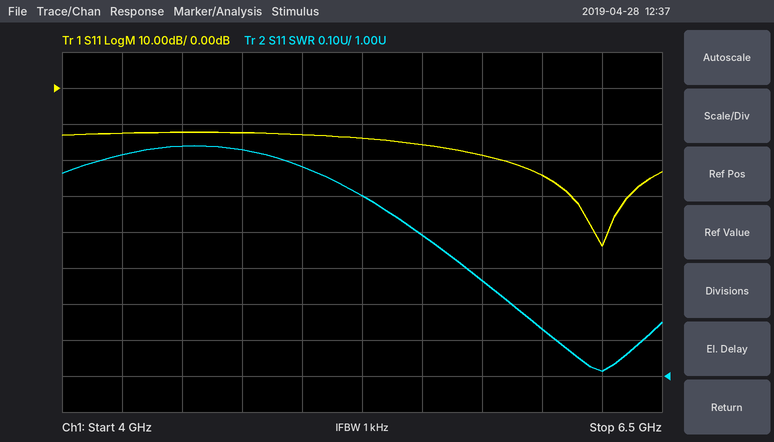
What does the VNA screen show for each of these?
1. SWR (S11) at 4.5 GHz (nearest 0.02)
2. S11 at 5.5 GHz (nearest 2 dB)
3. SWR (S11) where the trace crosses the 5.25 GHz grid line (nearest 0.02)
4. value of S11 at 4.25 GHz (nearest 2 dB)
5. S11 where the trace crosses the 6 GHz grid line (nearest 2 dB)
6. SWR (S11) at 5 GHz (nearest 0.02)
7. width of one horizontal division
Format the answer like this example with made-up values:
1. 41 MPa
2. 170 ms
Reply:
1. 1.64
2. -16 dB
3. 1.50
4. -12 dB
5. -24 dB
6. 1.58
7. 250 MHz
